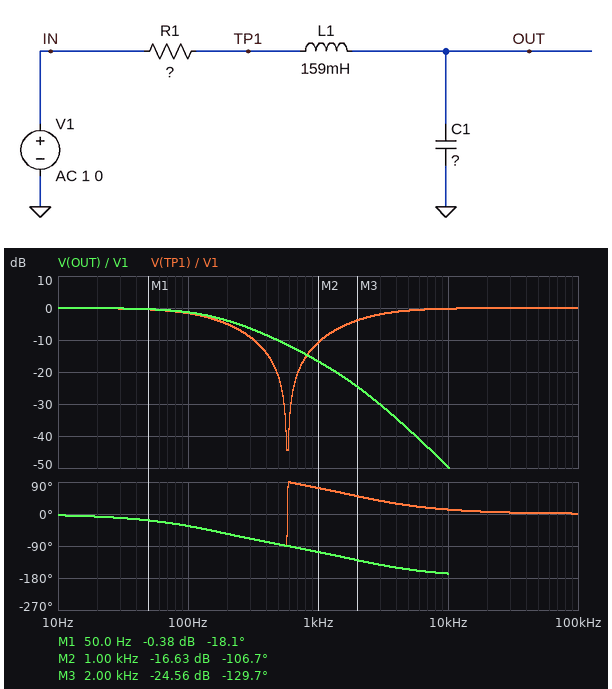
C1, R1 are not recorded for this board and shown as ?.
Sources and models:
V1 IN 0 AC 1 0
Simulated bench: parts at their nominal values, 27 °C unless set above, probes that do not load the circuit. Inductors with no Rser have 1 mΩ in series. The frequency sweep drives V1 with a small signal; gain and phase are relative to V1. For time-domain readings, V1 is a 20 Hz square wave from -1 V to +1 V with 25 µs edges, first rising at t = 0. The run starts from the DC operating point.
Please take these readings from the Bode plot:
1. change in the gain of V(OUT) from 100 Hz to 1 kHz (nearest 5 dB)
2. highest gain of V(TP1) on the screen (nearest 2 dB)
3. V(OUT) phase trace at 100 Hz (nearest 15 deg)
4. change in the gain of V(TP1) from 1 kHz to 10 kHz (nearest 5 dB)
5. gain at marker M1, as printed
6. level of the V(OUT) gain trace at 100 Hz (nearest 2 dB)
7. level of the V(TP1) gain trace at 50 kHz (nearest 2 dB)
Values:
-15 dB
0 dB
-30 deg
10 dB
-0.38 dB
-2 dB
0 dB
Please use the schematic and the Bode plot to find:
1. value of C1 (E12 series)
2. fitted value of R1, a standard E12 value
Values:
470 nF
2.2 kΩ
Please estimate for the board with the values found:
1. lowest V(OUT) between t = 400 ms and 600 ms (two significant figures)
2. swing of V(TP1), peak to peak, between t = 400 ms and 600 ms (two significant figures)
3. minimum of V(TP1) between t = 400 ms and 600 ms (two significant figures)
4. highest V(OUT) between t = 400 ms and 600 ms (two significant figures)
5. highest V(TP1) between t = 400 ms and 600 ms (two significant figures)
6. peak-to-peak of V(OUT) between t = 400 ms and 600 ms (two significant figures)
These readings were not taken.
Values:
-1.0 V
2.0 V
-1.0 V
1.0 V
1.0 V
2.0 V
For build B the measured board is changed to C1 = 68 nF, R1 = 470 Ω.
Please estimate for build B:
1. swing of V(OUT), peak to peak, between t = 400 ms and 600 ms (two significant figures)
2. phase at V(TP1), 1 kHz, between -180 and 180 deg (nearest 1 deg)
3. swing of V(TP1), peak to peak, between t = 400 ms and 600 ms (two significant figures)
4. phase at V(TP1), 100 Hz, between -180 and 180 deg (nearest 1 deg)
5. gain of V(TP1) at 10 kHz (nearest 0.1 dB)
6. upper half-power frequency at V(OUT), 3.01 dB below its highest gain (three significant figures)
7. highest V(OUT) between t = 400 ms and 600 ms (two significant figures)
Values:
4.5 V
-19 deg
2.6 V
-1 deg
0 dB
1.72 kHz
2.2 V
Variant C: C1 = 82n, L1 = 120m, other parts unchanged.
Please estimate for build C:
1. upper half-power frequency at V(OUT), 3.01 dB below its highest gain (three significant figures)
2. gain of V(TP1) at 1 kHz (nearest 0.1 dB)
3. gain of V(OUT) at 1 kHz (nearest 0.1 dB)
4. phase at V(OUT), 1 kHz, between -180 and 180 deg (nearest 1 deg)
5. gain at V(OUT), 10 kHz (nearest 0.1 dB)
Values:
1.18 kHz
-6.5 dB
-2.2 dB
-62 deg
-31.9 dB
